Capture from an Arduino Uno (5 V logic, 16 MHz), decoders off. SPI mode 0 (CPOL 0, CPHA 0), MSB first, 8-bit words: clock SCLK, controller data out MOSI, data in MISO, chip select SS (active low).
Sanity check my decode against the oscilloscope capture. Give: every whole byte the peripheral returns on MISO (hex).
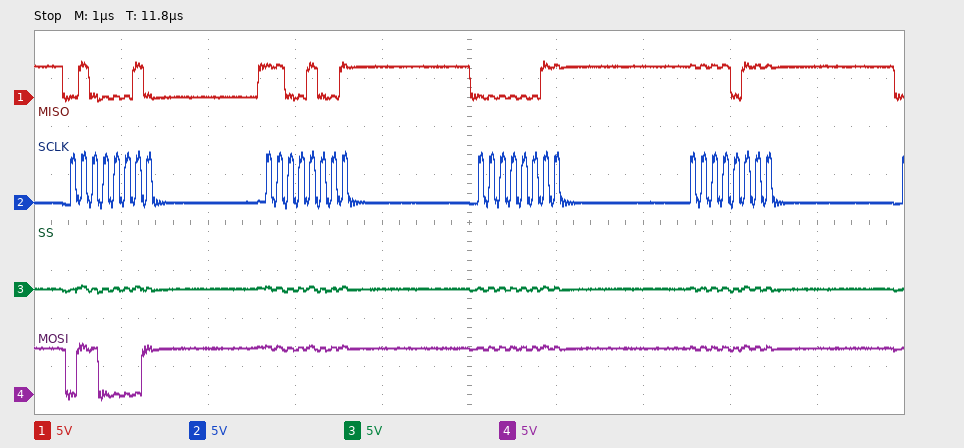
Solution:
0x42 0xC9 0x03 0xF7
